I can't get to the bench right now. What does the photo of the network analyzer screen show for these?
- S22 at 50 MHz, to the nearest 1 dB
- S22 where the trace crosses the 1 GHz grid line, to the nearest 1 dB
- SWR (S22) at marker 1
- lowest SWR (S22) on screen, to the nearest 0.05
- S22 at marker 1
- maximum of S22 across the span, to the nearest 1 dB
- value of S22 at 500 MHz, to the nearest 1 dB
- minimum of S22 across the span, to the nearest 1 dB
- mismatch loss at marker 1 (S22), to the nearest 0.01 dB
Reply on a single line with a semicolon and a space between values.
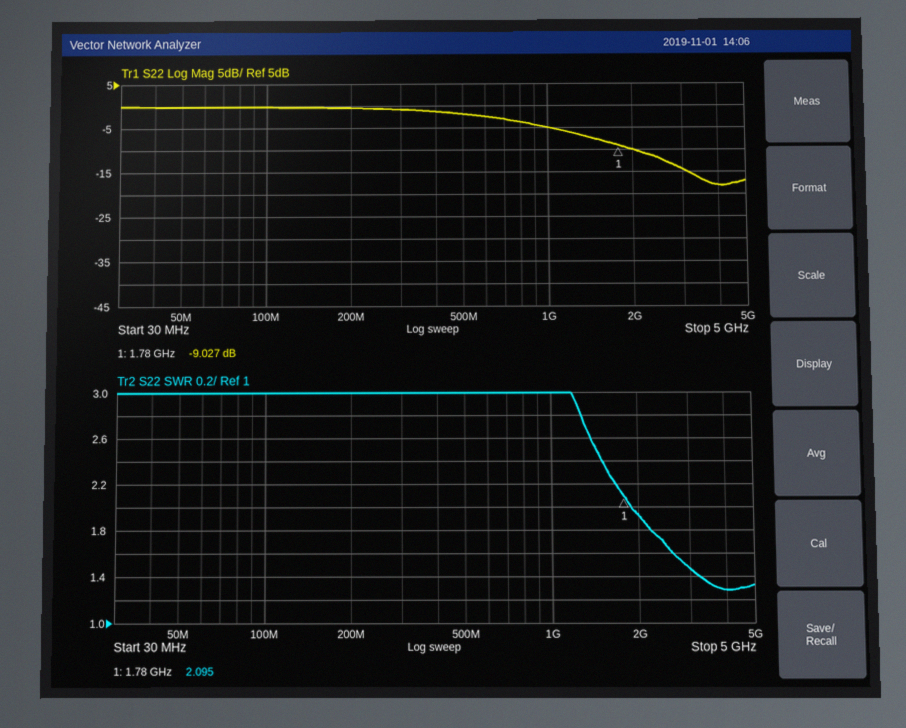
0 dB; -5 dB; 2.095; 1.30; -9.027 dB; 0 dB; -2 dB; -18 dB; 0.58 dB
